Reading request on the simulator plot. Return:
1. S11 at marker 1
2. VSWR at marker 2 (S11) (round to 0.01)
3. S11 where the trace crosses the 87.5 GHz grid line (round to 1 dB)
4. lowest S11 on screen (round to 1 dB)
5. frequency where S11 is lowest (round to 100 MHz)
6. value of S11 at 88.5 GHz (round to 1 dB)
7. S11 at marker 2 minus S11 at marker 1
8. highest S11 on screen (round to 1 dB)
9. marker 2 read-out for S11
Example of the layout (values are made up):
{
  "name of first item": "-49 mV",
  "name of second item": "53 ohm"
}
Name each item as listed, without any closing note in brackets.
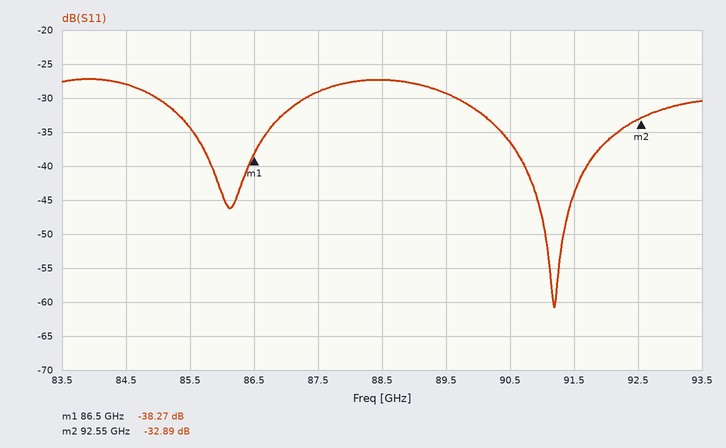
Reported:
{
  "S11 at marker 1": "-38.27 dB",
  "VSWR at marker 2 (S11)": "1.05",
  "S11 where the trace crosses the 87.5 GHz grid line": "-29 dB",
  "lowest S11 on screen": "-61 dB",
  "frequency where S11 is lowest": "91.2 GHz",
  "value of S11 at 88.5 GHz": "-27 dB",
  "S11 at marker 2 minus S11 at marker 1": "5.38 dB",
  "highest S11 on screen": "-27 dB",
  "marker 2 read-out for S11": "-32.89 dB"
}
